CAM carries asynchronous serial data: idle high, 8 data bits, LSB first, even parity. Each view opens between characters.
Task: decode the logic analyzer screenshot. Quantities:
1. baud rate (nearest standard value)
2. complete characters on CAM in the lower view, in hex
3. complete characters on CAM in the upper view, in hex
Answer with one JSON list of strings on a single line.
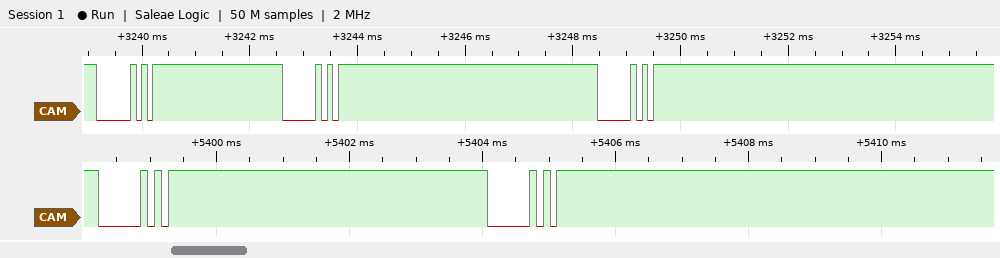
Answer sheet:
["9600 baud", "A0, A0", "A0, A0, A0"]
